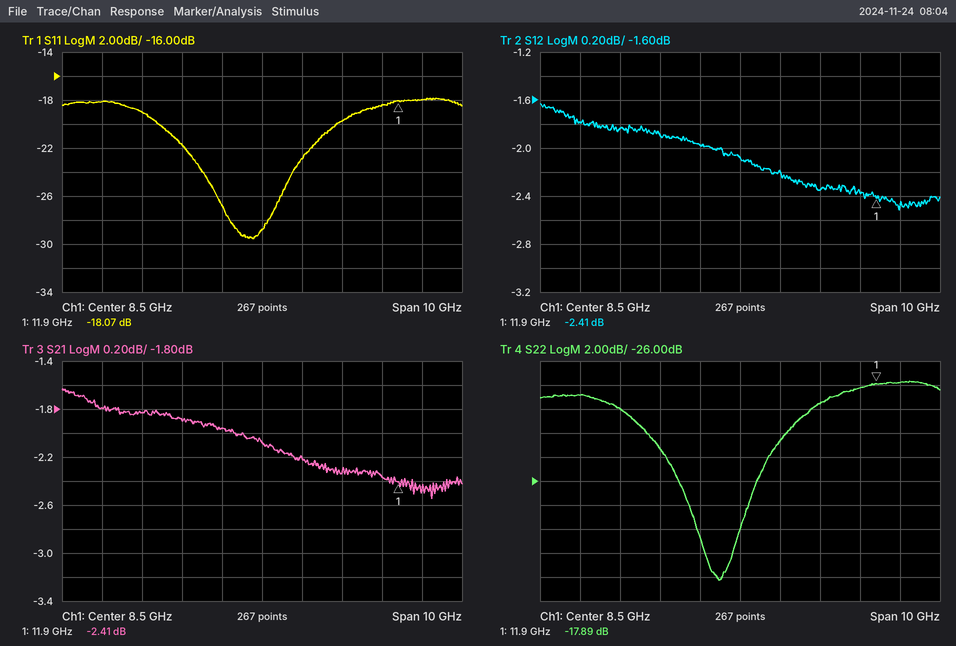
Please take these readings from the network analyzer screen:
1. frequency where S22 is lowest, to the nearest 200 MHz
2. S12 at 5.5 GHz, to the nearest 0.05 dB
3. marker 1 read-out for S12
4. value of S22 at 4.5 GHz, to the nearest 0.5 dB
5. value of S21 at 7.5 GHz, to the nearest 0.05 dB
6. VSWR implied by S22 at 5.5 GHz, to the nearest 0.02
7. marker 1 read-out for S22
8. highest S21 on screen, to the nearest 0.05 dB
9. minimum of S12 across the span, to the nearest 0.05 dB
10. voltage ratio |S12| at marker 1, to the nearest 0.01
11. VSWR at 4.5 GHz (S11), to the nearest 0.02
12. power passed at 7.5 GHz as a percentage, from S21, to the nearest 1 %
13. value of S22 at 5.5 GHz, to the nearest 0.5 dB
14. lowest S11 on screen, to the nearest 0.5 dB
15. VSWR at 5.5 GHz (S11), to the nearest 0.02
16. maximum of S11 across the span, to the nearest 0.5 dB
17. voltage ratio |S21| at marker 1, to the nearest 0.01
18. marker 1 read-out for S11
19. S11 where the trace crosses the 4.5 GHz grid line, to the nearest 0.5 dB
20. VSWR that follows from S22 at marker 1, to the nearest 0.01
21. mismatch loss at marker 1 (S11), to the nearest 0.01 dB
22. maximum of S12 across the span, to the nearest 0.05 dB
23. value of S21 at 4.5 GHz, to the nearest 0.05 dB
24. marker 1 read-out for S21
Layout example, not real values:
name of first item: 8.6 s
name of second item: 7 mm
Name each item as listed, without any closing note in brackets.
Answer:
frequency where S22 is lowest, to the nearest 200 MHz: 8.0 GHz
S12 at 5.5 GHz, to the nearest 0.05 dB: -1.85 dB
marker 1 read-out for S12: -2.41 dB
value of S22 at 4.5 GHz, to the nearest 0.5 dB: -19.0 dB
value of S21 at 7.5 GHz, to the nearest 0.05 dB: -1.95 dB
VSWR implied by S22 at 5.5 GHz, to the nearest 0.02: 1.22
marker 1 read-out for S22: -17.89 dB
highest S21 on screen, to the nearest 0.05 dB: -1.65 dB
minimum of S12 across the span, to the nearest 0.05 dB: -2.50 dB
voltage ratio |S12| at marker 1, to the nearest 0.01: 0.76
VSWR at 4.5 GHz (S11), to the nearest 0.02: 1.28
power passed at 7.5 GHz as a percentage, from S21, to the nearest 1 %: 64 %
value of S22 at 5.5 GHz, to the nearest 0.5 dB: -20.0 dB
lowest S11 on screen, to the nearest 0.5 dB: -29.5 dB
VSWR at 5.5 GHz (S11), to the nearest 0.02: 1.26
maximum of S11 across the span, to the nearest 0.5 dB: -18.0 dB
voltage ratio |S21| at marker 1, to the nearest 0.01: 0.76
marker 1 read-out for S11: -18.07 dB
S11 where the trace crosses the 4.5 GHz grid line, to the nearest 0.5 dB: -18.0 dB
VSWR that follows from S22 at marker 1, to the nearest 0.01: 1.29
mismatch loss at marker 1 (S11), to the nearest 0.01 dB: 0.07 dB
maximum of S12 across the span, to the nearest 0.05 dB: -1.65 dB
value of S21 at 4.5 GHz, to the nearest 0.05 dB: -1.80 dB
marker 1 read-out for S21: -2.41 dB
